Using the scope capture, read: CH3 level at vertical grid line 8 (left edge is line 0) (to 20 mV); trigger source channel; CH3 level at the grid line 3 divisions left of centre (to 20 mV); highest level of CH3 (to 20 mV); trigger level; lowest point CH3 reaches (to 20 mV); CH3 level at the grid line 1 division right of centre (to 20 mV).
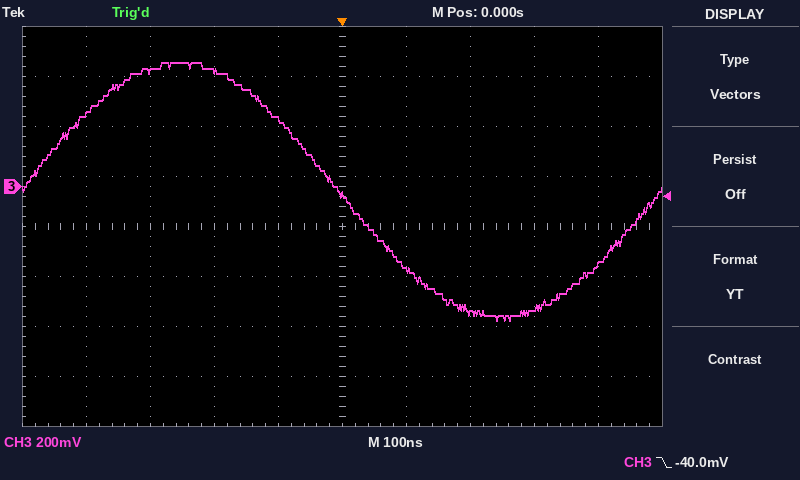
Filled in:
-480 mV
CH3
460 mV
500 mV
-40.0 mV
-540 mV
-340 mV
